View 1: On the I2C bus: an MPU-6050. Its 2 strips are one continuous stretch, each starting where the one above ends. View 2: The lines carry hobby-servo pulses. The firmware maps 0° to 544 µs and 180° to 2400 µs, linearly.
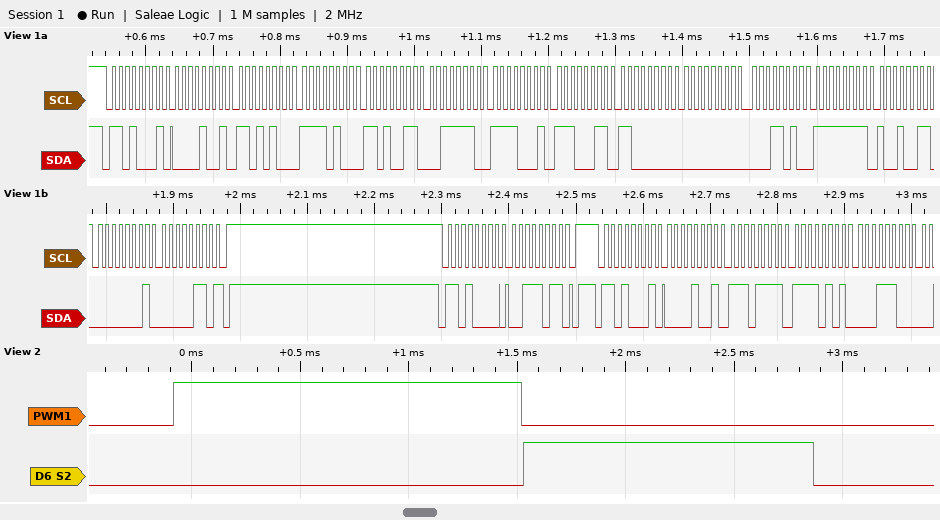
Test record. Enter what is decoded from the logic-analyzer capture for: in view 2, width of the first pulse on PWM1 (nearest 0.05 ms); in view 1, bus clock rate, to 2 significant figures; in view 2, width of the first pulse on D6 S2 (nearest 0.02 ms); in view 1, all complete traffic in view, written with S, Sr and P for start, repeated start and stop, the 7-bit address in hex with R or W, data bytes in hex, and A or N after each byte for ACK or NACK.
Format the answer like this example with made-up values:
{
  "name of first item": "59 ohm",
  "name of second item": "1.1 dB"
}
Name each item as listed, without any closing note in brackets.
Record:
{
  "in view 2, width of the first pulse on PWM1": "1.60 ms",
  "in view 1, bus clock rate, to 2 significant figures": "100 kHz",
  "in view 2, width of the first pulse on D6 S2": "1.34 ms",
  "in view 1, all complete traffic in view, written with S, Sr and P for start, repeated start and stop, the 7-bit address in hex with R or W, data bytes in hex, and A or N after each byte for ACK or NACK": "S 68R A 09 A D4 A F4 A D3 A 3E A F1 A E3 A C0 A 00 A 1A A FF A 93 A 01 A 06 N P S 68W A 3B A P S 68R A 09 A EF A F5 A 1C A"
}
